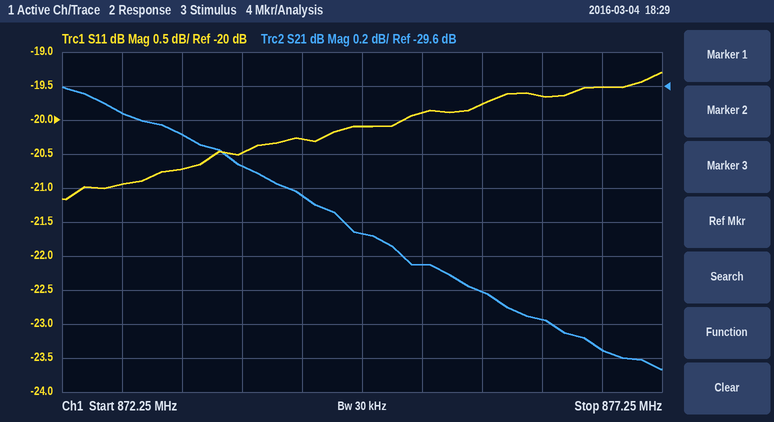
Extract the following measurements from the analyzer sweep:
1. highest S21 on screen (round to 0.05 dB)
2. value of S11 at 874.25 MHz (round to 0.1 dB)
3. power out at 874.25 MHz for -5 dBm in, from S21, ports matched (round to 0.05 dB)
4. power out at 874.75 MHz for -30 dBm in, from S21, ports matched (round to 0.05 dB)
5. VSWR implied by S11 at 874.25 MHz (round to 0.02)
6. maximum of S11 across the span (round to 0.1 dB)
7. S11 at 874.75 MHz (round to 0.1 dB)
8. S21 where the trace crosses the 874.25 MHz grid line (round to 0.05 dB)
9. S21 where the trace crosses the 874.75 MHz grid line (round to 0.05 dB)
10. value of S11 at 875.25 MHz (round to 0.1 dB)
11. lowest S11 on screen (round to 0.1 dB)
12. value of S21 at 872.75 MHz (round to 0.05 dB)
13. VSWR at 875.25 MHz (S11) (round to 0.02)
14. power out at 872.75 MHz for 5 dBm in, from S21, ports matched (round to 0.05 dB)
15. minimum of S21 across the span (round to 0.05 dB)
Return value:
-29.60 dB
-20.3 dB
-35.25 dBm
-60.45 dBm
1.22
-19.3 dB
-20.1 dB
-30.25 dB
-30.45 dB
-19.9 dB
-21.2 dB
-29.75 dB
1.22
-24.75 dBm
-31.25 dB
